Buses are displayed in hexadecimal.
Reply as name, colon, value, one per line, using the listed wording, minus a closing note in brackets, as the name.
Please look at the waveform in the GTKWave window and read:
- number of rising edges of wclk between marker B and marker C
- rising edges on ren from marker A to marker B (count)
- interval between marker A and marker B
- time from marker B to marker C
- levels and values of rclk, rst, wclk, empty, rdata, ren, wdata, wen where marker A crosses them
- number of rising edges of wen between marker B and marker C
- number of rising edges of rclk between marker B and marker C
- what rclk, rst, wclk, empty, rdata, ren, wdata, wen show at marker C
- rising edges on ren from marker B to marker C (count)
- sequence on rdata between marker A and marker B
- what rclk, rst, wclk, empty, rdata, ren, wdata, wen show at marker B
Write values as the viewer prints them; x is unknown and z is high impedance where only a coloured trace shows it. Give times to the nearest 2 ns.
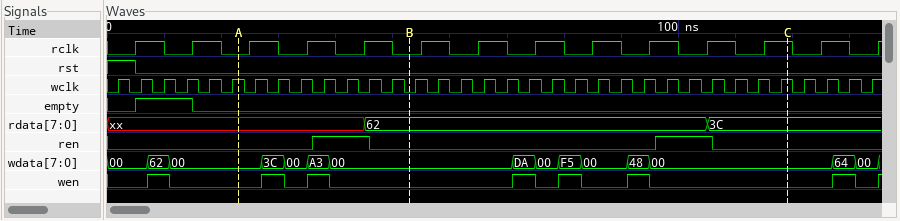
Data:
number of rising edges of wclk between marker B and marker C: 17
rising edges on ren from marker A to marker B: 1
interval between marker A and marker B: 30 ns
time from marker B to marker C: 66 ns
levels and values of rclk, rst, wclk, empty, rdata, ren, wdata, wen where marker A crosses them: rclk=0, rst=0, wclk=1, empty=0, rdata=xx, ren=0, wdata=00, wen=0
number of rising edges of wen between marker B and marker C: 3
number of rising edges of rclk between marker B and marker C: 7
what rclk, rst, wclk, empty, rdata, ren, wdata, wen show at marker C: rclk=1, rst=0, wclk=1, empty=0, rdata=3C, ren=0, wdata=00, wen=0
rising edges on ren from marker B to marker C: 1
sequence on rdata between marker A and marker B: xx, 62
what rclk, rst, wclk, empty, rdata, ren, wdata, wen show at marker B: rclk=0, rst=0, wclk=0, empty=0, rdata=62, ren=0, wdata=00, wen=0
